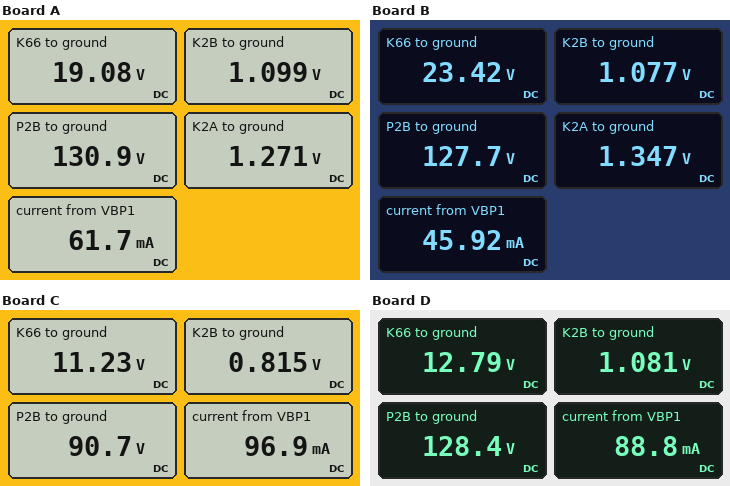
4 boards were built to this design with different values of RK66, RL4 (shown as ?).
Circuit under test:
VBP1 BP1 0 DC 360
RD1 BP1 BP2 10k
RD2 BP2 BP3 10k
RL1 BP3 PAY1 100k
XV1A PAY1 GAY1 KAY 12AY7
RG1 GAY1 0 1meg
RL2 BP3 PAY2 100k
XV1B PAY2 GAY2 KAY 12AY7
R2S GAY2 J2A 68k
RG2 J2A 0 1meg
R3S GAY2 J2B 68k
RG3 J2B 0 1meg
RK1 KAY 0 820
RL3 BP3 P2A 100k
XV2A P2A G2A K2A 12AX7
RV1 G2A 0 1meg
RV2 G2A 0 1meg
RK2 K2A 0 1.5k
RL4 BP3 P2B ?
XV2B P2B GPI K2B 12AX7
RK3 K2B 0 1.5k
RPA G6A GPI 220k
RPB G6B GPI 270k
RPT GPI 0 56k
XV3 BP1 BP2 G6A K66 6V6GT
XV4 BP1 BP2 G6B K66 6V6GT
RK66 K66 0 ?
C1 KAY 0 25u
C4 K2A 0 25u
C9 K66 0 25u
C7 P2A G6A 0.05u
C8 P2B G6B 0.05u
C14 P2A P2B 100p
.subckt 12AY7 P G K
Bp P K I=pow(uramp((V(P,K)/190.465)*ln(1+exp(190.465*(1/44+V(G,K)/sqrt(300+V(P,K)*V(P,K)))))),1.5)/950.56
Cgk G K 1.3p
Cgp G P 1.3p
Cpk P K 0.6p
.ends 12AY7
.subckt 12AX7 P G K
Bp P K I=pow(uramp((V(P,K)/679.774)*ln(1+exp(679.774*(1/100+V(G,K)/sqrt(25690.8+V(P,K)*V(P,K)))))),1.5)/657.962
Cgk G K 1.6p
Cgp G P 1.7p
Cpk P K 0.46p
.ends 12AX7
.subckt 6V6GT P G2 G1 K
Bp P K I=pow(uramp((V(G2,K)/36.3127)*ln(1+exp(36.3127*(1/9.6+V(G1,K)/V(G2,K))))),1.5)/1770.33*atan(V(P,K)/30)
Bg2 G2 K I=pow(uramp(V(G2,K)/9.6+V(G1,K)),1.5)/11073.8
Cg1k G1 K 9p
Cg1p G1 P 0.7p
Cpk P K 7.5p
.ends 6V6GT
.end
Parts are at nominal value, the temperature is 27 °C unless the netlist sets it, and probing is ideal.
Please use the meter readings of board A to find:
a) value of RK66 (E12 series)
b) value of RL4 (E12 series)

330 Ω
150 kΩ
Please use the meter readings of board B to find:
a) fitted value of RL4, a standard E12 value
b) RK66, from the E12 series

180 kΩ
560 Ω
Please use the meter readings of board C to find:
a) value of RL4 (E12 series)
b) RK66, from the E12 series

220 kΩ
120 Ω
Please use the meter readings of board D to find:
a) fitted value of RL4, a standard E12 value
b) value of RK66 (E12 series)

120 kΩ
150 Ω
